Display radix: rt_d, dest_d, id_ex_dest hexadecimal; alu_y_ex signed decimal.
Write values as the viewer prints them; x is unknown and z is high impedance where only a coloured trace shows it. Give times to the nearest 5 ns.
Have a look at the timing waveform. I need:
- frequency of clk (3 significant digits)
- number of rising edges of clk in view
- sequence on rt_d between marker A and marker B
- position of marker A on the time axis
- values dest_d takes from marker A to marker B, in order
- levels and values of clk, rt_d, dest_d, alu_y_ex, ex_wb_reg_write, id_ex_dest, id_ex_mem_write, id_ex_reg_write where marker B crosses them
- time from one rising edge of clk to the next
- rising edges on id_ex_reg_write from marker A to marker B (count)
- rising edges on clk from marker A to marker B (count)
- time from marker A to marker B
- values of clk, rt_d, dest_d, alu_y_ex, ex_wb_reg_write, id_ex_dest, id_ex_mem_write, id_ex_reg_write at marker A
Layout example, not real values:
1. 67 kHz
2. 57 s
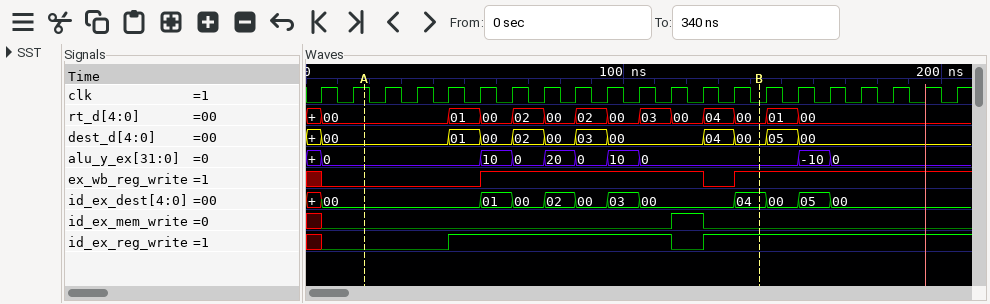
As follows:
1. 100 MHz
2. 21
3. 00, 01, 00, 02, 00, 02, 00, 03, 00, 04, 00
4. 20 ns
5. 00, 01, 00, 02, 00, 03, 00, 04, 00
6. clk=0, rt_d=00, dest_d=00, alu_y_ex=0, ex_wb_reg_write=1, id_ex_dest=04, id_ex_mem_write=0, id_ex_reg_write=1
7. 10 ns
8. 2
9. 12
10. 125 ns
11. clk=1, rt_d=00, dest_d=00, alu_y_ex=0, ex_wb_reg_write=0, id_ex_dest=00, id_ex_mem_write=0, id_ex_reg_write=0
